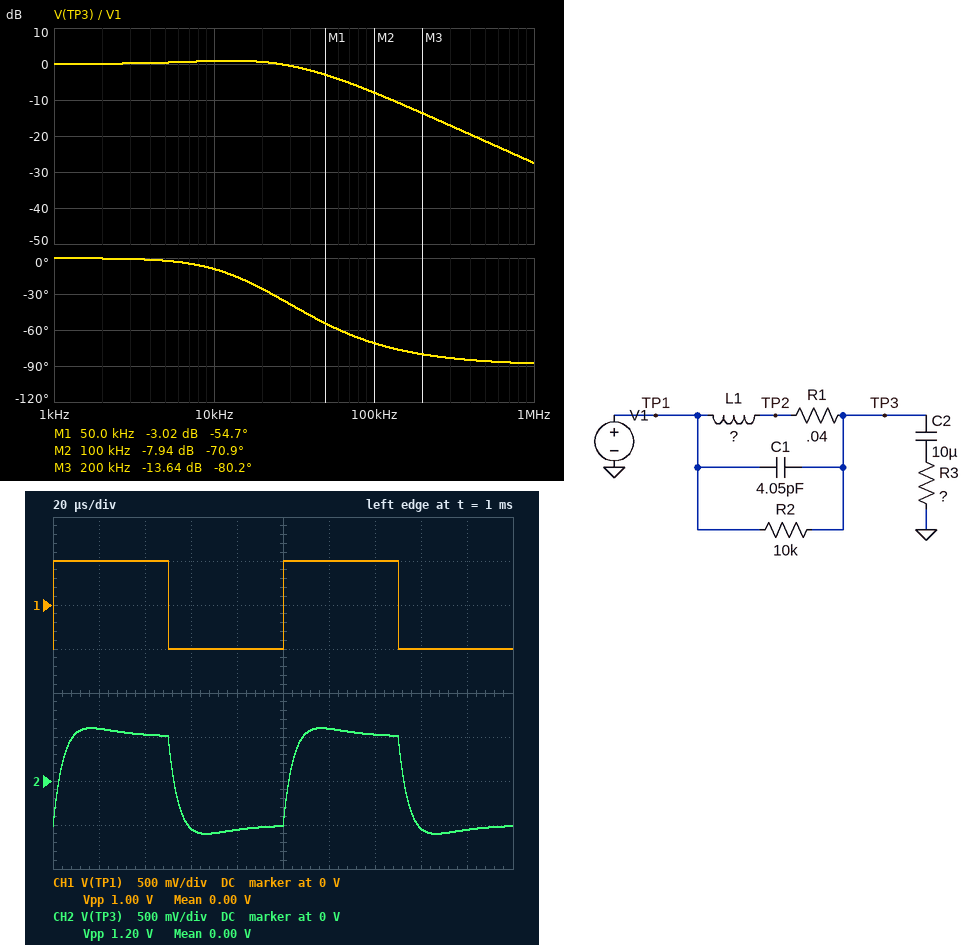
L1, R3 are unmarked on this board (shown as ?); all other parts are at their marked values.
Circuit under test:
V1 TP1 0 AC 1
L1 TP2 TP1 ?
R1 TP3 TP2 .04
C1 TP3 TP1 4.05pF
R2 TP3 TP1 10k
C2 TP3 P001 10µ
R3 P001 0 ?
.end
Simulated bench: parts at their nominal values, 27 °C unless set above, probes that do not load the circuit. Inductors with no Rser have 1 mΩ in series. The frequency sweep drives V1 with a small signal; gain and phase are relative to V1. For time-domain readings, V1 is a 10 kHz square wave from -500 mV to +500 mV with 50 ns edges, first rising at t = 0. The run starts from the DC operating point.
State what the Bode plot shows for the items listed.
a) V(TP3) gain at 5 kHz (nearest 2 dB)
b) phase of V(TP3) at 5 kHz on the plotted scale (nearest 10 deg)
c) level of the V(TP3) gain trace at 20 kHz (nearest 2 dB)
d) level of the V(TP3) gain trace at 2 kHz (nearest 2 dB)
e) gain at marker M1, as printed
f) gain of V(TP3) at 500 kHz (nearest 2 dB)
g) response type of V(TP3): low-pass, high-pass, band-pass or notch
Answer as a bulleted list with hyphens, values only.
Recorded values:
- 0 dB
- 0 deg
- 0 dB
- 0 dB
- -3.02 dB
- -22 dB
- low-pass
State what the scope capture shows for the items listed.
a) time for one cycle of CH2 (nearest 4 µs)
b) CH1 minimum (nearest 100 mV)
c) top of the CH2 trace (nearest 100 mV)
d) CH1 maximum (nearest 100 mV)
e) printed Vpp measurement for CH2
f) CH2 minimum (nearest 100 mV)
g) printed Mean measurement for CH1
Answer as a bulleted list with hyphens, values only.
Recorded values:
- 100 µs
- -500 mV
- 600 mV
- 500 mV
- 1.20 V
- -600 mV
- 0.00 V
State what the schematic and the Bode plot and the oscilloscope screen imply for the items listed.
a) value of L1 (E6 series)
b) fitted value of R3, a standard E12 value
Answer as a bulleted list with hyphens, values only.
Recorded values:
- 6.8 µH
- 1.8 Ω
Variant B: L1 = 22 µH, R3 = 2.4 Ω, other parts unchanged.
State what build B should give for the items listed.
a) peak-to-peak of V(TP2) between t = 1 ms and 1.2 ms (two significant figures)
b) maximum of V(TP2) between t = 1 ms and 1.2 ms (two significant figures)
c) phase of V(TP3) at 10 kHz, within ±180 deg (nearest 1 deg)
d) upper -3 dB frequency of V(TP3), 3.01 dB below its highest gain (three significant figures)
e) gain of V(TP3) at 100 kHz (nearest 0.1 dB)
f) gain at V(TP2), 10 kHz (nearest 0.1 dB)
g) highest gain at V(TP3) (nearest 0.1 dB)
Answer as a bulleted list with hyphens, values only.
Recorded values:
- 1.3 V
- 660 mV
- -29 deg
- 18.7 kHz
- -15.2 dB
- 1.5 dB
- 1.6 dB
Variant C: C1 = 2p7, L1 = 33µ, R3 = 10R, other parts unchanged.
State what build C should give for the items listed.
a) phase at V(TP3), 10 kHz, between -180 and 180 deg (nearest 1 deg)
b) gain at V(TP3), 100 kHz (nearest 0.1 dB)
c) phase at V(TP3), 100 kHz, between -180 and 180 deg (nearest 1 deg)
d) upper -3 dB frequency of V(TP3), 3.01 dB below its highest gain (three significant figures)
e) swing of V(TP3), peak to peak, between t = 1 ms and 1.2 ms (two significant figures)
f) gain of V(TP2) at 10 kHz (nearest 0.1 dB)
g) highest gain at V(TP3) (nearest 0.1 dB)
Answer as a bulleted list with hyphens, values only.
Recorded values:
- -12 deg
- -7.2 dB
- -65 deg
- 47.5 kHz
- 1.0 V
- 0.1 dB
- 0.2 dB
